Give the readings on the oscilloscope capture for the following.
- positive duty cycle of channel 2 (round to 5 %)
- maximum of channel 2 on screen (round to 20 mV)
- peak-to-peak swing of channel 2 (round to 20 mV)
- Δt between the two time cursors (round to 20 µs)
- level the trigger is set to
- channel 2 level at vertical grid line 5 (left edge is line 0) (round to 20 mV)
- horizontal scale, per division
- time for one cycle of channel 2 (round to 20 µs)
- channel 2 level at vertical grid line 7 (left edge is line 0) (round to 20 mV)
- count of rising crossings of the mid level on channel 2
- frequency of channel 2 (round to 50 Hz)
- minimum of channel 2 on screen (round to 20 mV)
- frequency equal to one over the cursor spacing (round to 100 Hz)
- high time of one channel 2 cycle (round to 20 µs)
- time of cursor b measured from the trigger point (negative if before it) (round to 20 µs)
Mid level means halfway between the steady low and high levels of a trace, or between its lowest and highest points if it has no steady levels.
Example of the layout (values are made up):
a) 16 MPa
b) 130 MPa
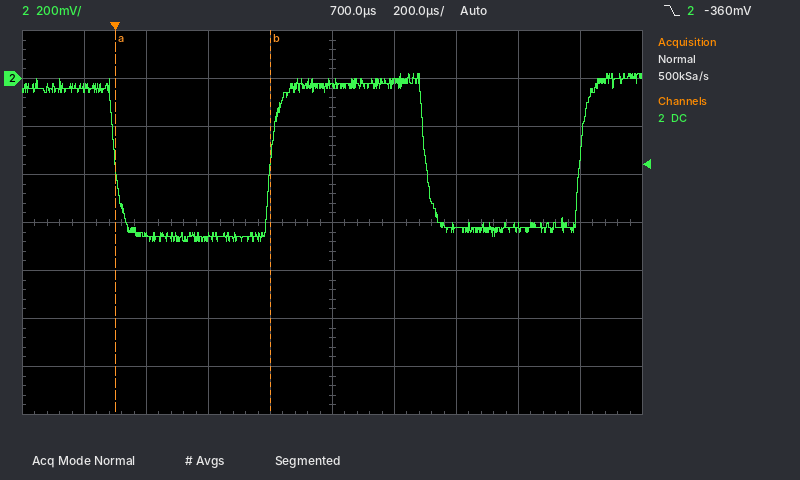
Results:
a) 50 %
b) 20 mV
c) 700 mV
d) 500 µs
e) -360 mV
f) -20 mV
g) 200 µs
h) 1.00 ms
i) -620 mV
j) 2
k) 1.00 kHz
l) -680 mV
m) 2.0 kHz
n) 500 µs
o) +500 µs
